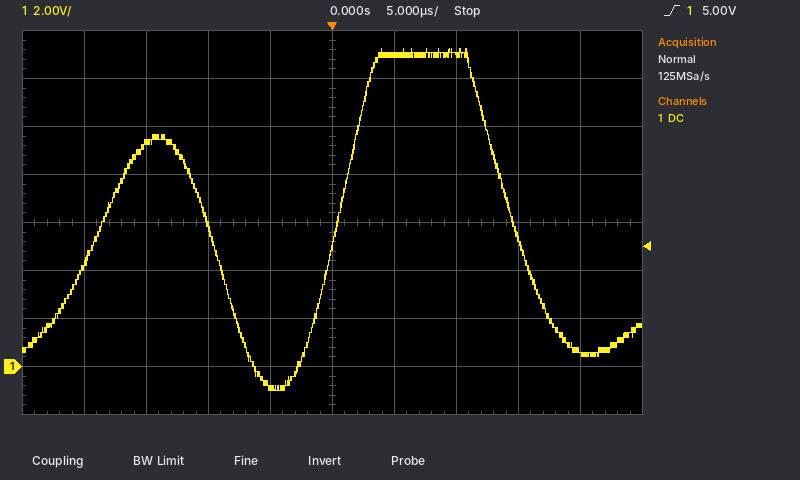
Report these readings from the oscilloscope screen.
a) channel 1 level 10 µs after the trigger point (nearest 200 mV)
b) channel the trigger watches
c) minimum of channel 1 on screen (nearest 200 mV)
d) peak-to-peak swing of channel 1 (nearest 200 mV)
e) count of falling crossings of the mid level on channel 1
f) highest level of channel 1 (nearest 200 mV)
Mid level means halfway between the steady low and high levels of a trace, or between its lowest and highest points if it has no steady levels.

13.0 V
channel 1
-1.0 V
14.2 V
2
13.2 V
